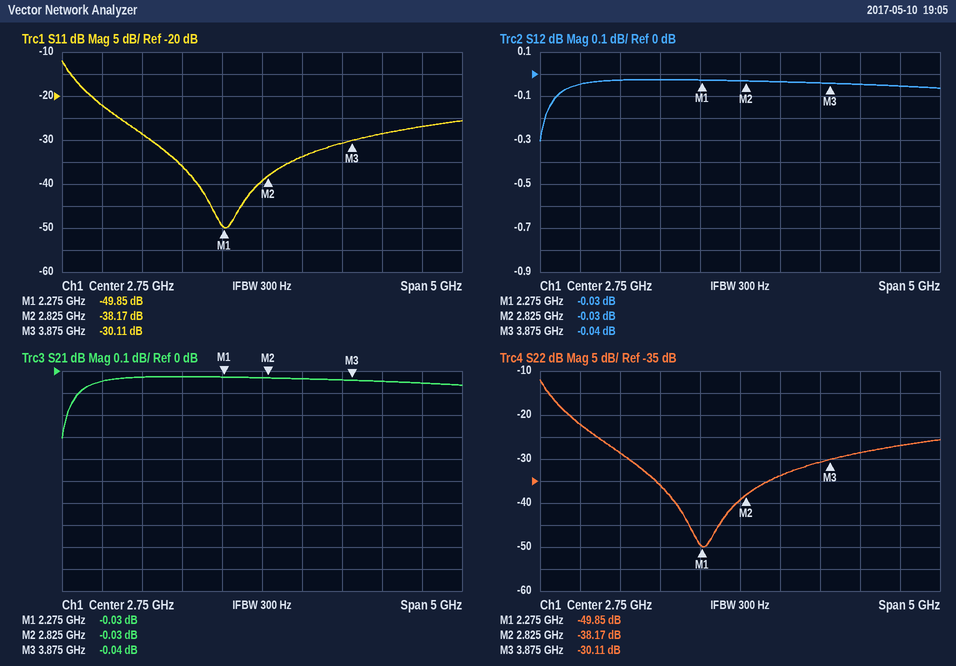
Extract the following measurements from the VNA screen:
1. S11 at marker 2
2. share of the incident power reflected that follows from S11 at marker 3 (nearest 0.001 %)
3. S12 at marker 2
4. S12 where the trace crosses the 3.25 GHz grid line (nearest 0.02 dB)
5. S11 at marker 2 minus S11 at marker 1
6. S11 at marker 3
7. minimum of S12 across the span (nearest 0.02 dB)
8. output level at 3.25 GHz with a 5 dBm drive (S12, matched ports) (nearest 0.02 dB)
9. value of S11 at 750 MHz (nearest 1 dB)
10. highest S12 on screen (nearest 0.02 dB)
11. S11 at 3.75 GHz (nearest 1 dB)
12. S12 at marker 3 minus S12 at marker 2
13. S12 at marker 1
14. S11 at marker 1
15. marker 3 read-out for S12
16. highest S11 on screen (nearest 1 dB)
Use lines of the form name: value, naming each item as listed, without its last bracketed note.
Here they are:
S11 at marker 2: -38.17 dB
share of the incident power reflected that follows from S11 at marker 3: 0.097 %
S12 at marker 2: -0.03 dB
S12 where the trace crosses the 3.25 GHz grid line: -0.04 dB
S11 at marker 2 minus S11 at marker 1: 11.68 dB
S11 at marker 3: -30.11 dB
minimum of S12 across the span: -0.30 dB
output level at 3.25 GHz with a 5 dBm drive (S12, matched ports): 4.96 dBm
value of S11 at 750 MHz: -22 dB
highest S12 on screen: -0.02 dB
S11 at 3.75 GHz: -31 dB
S12 at marker 3 minus S12 at marker 2: -0.01 dB
S12 at marker 1: -0.03 dB
S11 at marker 1: -49.85 dB
marker 3 read-out for S12: -0.04 dB
highest S11 on screen: -12 dB
